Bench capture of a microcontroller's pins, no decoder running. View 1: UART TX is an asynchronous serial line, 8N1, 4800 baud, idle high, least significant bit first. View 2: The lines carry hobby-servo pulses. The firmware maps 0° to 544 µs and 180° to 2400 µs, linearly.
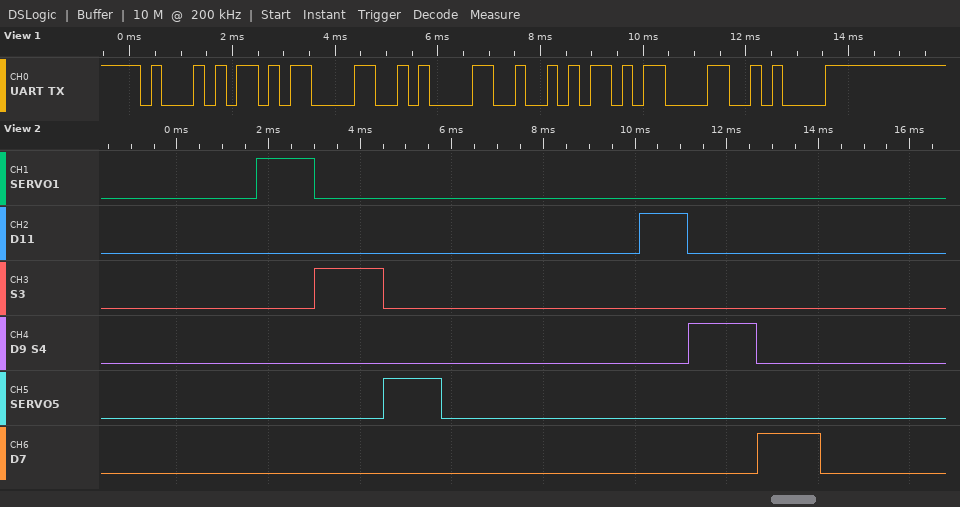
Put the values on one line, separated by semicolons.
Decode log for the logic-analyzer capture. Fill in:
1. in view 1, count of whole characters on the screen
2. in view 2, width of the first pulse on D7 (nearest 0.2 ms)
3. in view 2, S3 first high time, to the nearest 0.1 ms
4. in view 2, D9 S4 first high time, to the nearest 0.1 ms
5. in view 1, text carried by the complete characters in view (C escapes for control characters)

6; 1.4 ms; 1.5 ms; 1.5 ms; "Q\r\nR\r\n"
